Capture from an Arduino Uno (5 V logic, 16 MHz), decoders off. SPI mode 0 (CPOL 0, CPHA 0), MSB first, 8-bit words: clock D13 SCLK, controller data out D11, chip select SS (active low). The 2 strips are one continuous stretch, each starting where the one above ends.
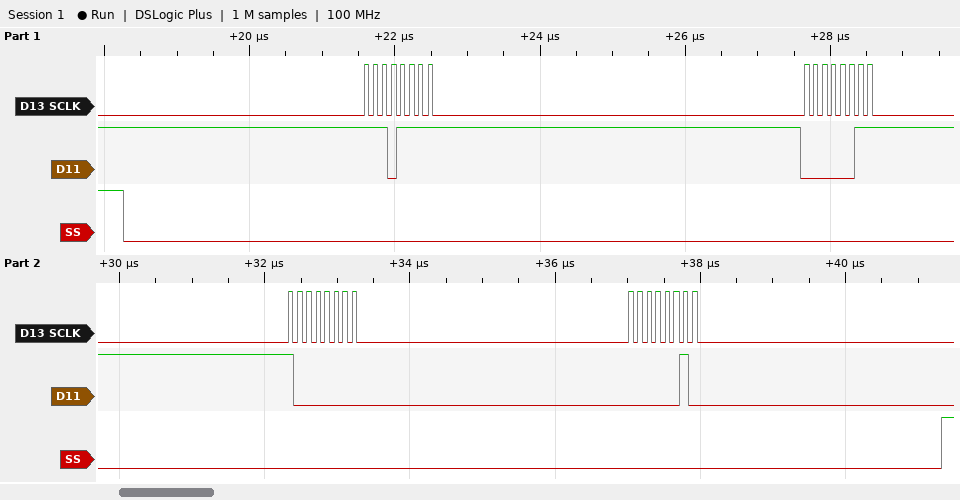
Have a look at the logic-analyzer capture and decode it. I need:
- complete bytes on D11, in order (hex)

EF 03 80 02
